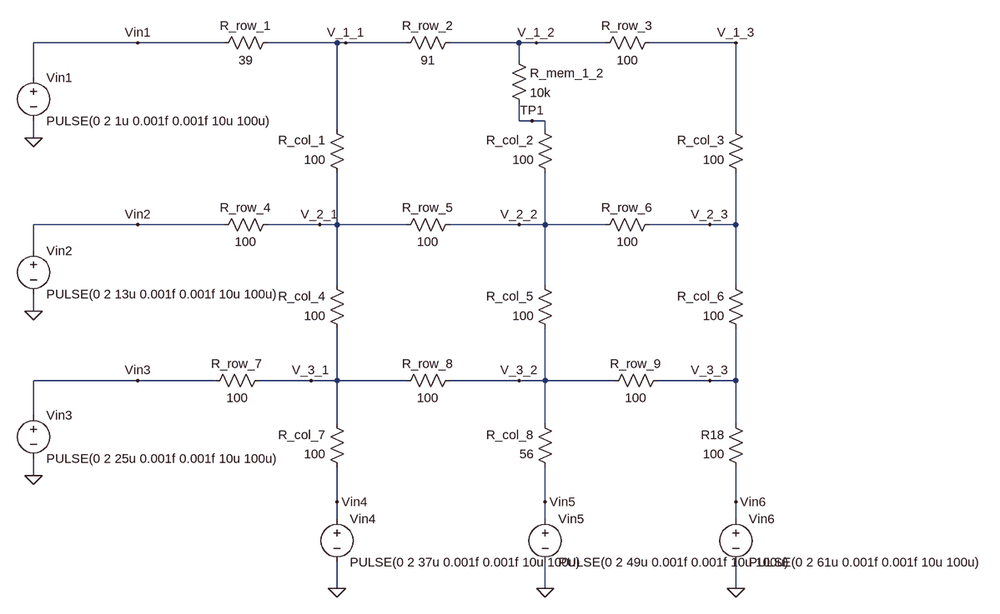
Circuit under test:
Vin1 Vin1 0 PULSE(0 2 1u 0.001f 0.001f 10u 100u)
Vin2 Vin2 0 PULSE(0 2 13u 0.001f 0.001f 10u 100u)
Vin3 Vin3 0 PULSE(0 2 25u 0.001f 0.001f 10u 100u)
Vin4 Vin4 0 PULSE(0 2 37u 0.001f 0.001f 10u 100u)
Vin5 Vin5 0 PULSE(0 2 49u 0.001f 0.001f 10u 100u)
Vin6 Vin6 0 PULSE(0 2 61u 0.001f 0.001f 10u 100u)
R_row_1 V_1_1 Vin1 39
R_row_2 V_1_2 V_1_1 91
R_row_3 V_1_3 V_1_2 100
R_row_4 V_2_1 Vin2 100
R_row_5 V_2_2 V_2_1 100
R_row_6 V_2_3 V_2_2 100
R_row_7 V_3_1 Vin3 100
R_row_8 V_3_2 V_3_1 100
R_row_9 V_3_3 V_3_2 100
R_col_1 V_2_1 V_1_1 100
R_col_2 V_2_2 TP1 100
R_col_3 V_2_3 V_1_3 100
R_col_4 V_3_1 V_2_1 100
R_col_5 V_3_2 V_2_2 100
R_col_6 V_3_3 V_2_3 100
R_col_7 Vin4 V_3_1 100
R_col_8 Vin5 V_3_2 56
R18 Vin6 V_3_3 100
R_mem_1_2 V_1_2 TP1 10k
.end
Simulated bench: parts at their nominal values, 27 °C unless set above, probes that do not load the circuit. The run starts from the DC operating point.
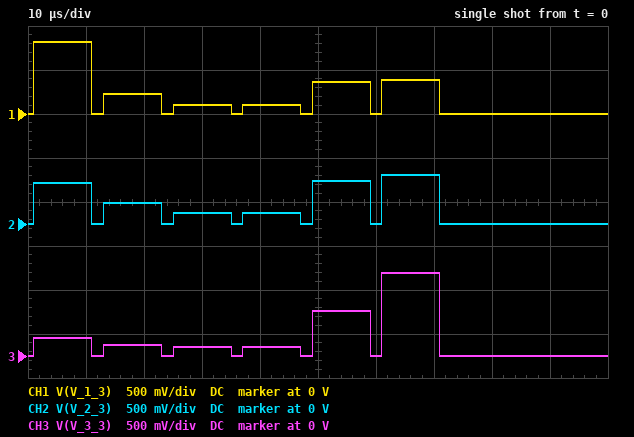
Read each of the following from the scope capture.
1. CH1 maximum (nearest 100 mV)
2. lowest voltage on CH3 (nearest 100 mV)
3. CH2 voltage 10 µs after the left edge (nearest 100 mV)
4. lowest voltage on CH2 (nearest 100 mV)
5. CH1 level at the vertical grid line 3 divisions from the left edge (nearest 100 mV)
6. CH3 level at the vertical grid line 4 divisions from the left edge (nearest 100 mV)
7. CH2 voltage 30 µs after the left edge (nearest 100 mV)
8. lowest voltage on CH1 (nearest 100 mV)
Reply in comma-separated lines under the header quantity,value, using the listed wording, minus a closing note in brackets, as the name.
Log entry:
quantity,value
CH1 maximum,800 mV
lowest voltage on CH3,0 V
CH2 voltage 10 µs after the left edge,500 mV
lowest voltage on CH2,0 V
CH1 level at the vertical grid line 3 divisions from the left edge,100 mV
CH3 level at the vertical grid line 4 divisions from the left edge,100 mV
CH2 voltage 30 µs after the left edge,100 mV
lowest voltage on CH1,0 V
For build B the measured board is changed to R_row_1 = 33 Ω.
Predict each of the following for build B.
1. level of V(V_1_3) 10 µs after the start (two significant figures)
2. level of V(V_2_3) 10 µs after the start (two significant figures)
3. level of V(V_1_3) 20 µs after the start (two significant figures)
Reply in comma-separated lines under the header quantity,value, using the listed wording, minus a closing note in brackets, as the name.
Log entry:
quantity,value
level of V(V_1_3) 10 µs after the start,850 mV
level of V(V_2_3) 10 µs after the start,490 mV
level of V(V_1_3) 20 µs after the start,210 mV
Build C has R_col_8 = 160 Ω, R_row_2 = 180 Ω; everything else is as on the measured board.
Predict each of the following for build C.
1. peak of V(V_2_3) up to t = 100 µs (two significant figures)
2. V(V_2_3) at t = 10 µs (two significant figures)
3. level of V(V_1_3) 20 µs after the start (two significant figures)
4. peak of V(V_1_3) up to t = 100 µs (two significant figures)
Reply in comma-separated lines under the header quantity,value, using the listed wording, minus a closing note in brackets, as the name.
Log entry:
quantity,value
peak of V(V_2_3) up to t = 100 µs,650 mV
V(V_2_3) at t = 10 µs,450 mV
level of V(V_1_3) 20 µs after the start,260 mV
peak of V(V_1_3) up to t = 100 µs,730 mV
